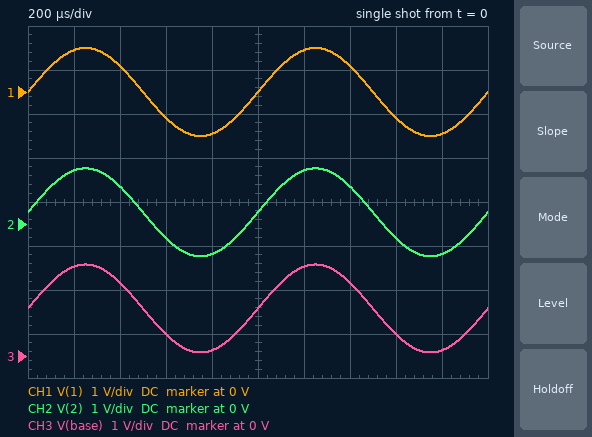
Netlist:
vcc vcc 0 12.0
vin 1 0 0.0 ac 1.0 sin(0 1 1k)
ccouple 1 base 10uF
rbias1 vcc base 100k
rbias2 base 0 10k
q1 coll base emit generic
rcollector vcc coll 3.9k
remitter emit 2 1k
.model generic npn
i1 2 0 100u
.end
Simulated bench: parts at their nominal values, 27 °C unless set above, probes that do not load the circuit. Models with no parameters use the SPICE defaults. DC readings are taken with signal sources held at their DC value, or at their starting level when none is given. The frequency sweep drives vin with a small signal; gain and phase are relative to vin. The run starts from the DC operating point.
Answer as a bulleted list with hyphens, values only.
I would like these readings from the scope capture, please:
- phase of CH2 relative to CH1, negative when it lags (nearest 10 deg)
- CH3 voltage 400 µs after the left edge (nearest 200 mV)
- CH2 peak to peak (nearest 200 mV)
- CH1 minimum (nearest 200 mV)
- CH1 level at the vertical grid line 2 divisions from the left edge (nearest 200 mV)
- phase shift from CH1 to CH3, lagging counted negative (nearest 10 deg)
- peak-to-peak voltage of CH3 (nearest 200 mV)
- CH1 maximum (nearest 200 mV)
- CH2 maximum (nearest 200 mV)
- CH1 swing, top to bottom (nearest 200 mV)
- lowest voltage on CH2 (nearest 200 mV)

- 0 deg
- 1.6 V
- 2.0 V
- -1.0 V
- 600 mV
- 0 deg
- 2.0 V
- 1.0 V
- 1.2 V
- 2.0 V
- -800 mV
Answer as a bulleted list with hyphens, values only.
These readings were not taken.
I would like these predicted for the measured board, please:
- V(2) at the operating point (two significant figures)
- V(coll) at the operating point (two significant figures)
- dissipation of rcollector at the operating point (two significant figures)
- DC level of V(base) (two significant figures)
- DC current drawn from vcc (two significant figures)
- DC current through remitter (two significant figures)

- 270 mV
- 12 V
- 38 µW
- 1.1 V
- 210 µA
- 100 µA
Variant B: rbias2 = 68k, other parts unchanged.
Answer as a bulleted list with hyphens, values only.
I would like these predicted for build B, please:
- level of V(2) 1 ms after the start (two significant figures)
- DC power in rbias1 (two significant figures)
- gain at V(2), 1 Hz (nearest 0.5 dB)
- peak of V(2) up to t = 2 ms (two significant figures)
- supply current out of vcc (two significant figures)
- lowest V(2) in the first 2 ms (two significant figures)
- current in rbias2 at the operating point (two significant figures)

- 4.0 V
- 520 µW
- -0.5 dB
- 5.0 V
- 170 µA
- 3.0 V
- 71 µA
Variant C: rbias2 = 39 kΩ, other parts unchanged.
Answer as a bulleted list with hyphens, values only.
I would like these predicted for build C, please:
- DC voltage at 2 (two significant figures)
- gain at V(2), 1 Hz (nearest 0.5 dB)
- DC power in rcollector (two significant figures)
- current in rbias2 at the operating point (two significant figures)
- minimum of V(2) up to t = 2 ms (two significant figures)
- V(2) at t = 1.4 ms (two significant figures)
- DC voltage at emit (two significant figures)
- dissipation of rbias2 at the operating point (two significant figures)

- 2.5 V
- -1.0 dB
- 38 µW
- 86 µA
- 1.5 V
- 3.1 V
- 2.6 V
- 290 µW
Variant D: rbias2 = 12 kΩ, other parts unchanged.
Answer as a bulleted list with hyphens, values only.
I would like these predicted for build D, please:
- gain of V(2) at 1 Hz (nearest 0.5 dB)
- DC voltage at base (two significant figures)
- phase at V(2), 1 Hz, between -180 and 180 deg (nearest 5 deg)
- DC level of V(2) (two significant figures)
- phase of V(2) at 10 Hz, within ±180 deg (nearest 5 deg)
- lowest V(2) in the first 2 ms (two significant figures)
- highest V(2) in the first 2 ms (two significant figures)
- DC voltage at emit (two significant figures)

- -5.0 dB
- 1.3 V
- 55 deg
- 460 mV
- 10 deg
- -540 mV
- 1.5 V
- 560 mV
